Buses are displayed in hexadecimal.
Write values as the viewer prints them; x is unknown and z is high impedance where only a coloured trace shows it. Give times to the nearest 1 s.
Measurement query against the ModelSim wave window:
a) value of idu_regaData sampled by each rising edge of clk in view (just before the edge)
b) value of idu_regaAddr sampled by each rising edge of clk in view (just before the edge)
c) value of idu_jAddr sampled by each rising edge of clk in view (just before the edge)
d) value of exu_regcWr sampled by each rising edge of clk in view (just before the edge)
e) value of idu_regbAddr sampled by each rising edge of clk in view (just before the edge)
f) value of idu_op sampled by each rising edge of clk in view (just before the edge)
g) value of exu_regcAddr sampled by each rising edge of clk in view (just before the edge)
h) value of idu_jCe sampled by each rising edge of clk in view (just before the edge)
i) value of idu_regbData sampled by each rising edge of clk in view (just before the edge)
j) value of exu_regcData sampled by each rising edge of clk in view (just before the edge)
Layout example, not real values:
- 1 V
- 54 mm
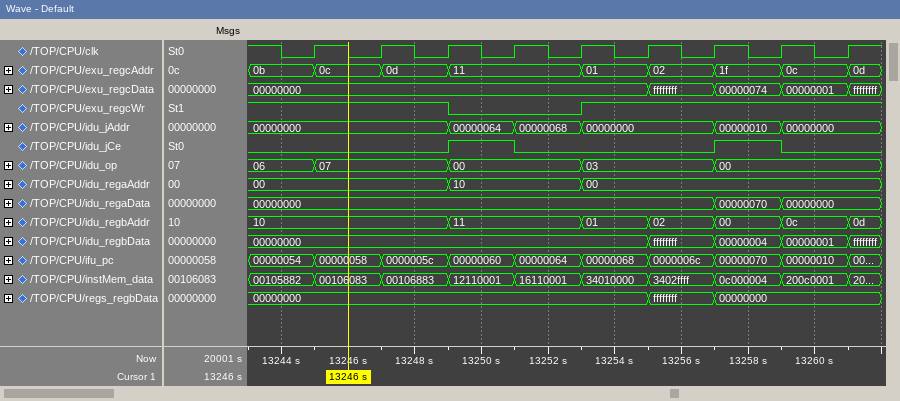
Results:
- 00000000, 00000000, 00000000, 00000000, 00000000, 00000000, 00000000, 00000070, 00000000
- 00, 00, 00, 10, 10, 00, 00, 00, 00
- 00000000, 00000000, 00000000, 00000064, 00000068, 00000000, 00000000, 00000010, 00000000
- 1 1 1 0 0 1 1 1 1
- 10, 10, 10, 11, 11, 01, 02, 00, 0c
- 06, 07, 07, 00, 00, 03, 03, 00, 00
- 0b, 0c, 0d, 11, 11, 01, 02, 1f, 0c
- 0 0 0 1 0 0 0 1 0
- 00000000, 00000000, 00000000, 00000000, 00000000, 00000000, ffffffff, 00000004, 00000001
- 00000000, 00000000, 00000000, 00000000, 00000000, 00000000, ffffffff, 00000074, 00000001
